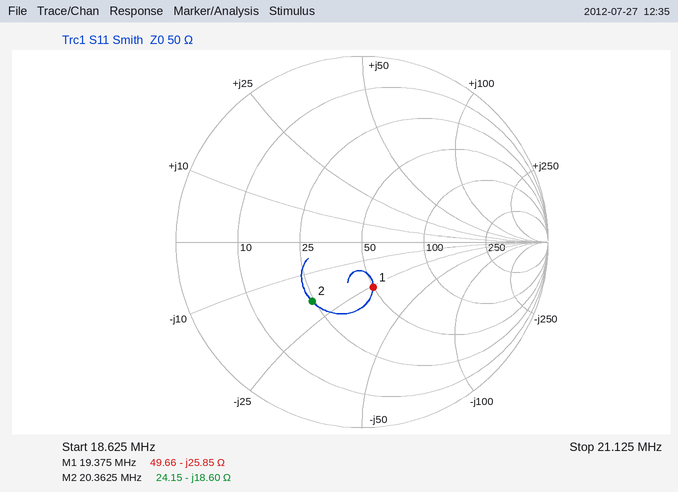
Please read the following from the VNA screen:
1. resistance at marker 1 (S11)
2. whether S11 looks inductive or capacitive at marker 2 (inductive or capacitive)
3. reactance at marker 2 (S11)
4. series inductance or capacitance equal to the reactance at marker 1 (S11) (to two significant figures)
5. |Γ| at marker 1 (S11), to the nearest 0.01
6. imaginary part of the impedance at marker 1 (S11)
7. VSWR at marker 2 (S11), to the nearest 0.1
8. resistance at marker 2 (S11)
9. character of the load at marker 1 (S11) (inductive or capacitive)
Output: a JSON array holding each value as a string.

["49.66 Ω", "capacitive", "-18.60 Ω", "320 pF", "0.25", "-25.85 Ω", "2.4", "24.15 Ω", "capacitive"]
